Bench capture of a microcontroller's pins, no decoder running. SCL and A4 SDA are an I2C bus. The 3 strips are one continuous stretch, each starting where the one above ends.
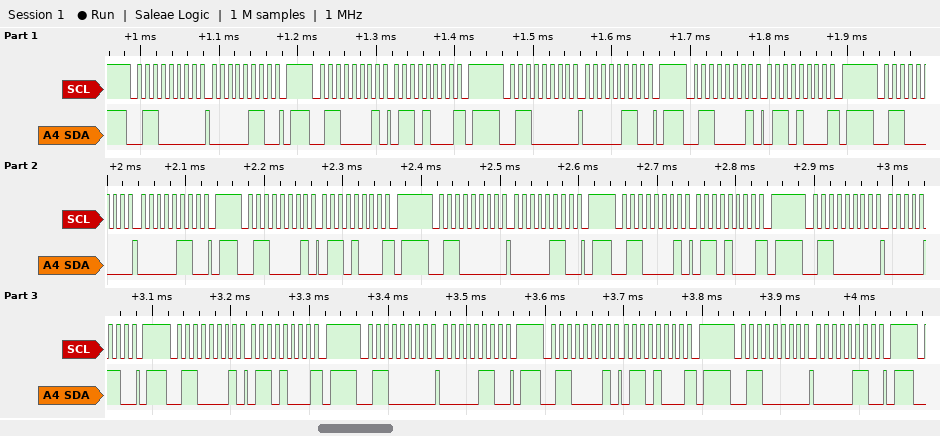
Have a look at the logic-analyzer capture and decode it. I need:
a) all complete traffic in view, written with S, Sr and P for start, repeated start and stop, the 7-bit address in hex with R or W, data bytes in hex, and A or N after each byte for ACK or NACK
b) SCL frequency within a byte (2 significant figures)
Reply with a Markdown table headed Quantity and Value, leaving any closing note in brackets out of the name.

| Quantity | Value |
|---|---|
| all complete traffic in view, written with S, Sr and P for start, repeated start and stop, the 7-bit address in hex with R or W, data bytes in hex, and A or N after each byte for ACK or NACK | S 30W A 06 A P S 30R A 68 N P S 30W A 06 A P S 30R A 68 N P S 30W A 06 A P S 30R A 68 N P S 30W A 06 A P S 30R A 68 N P S 30W A 06 A P S 30R A 68 N P S 30W A 06 A P S 30R A 68 N P S 30W A 06 A P |
| SCL frequency within a byte | 100 kHz |
